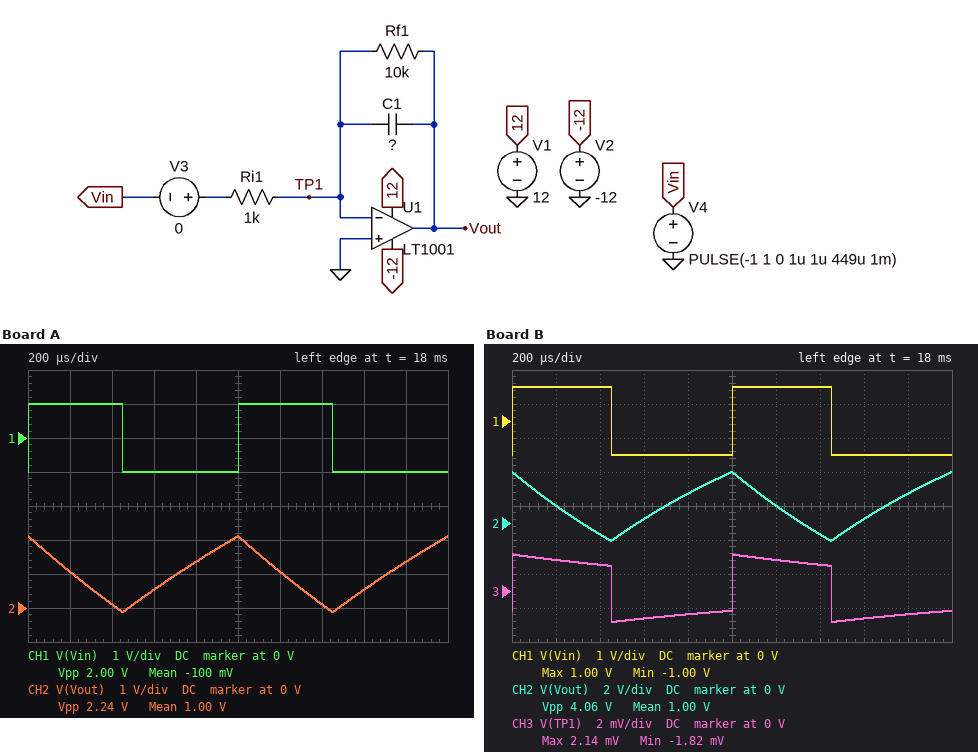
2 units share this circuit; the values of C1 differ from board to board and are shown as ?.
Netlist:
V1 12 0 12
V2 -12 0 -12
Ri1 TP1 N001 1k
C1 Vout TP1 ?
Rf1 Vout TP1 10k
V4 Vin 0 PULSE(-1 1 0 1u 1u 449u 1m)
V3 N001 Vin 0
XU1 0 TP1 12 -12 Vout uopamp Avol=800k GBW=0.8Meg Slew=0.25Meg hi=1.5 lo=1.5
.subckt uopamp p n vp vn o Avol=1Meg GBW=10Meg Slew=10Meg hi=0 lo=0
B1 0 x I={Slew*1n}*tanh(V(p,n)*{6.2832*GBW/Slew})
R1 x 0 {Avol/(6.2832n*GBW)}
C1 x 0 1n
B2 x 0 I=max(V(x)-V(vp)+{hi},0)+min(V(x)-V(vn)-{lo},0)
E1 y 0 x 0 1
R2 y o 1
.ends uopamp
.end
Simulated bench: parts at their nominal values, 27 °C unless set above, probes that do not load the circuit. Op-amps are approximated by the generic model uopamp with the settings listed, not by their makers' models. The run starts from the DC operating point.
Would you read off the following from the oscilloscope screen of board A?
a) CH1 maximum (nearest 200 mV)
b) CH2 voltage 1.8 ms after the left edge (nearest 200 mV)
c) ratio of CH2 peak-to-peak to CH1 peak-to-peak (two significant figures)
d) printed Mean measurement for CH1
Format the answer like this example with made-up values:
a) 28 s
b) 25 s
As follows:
a) 1.0 V
b) 1.4 V
c) 1.1
d) -100 mV
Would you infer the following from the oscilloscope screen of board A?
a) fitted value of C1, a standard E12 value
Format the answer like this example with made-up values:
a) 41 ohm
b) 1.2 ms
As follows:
a) 220 nF
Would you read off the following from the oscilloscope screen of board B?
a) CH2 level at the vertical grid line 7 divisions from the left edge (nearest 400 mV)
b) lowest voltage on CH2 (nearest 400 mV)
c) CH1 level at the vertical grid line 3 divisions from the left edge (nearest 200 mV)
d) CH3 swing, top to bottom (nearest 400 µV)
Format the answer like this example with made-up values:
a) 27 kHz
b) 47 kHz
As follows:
a) -800 mV
b) -1.2 V
c) -1.0 V
d) 4.0 mV
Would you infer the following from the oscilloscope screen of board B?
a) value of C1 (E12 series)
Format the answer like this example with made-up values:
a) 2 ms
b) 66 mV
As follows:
a) 120 nF
